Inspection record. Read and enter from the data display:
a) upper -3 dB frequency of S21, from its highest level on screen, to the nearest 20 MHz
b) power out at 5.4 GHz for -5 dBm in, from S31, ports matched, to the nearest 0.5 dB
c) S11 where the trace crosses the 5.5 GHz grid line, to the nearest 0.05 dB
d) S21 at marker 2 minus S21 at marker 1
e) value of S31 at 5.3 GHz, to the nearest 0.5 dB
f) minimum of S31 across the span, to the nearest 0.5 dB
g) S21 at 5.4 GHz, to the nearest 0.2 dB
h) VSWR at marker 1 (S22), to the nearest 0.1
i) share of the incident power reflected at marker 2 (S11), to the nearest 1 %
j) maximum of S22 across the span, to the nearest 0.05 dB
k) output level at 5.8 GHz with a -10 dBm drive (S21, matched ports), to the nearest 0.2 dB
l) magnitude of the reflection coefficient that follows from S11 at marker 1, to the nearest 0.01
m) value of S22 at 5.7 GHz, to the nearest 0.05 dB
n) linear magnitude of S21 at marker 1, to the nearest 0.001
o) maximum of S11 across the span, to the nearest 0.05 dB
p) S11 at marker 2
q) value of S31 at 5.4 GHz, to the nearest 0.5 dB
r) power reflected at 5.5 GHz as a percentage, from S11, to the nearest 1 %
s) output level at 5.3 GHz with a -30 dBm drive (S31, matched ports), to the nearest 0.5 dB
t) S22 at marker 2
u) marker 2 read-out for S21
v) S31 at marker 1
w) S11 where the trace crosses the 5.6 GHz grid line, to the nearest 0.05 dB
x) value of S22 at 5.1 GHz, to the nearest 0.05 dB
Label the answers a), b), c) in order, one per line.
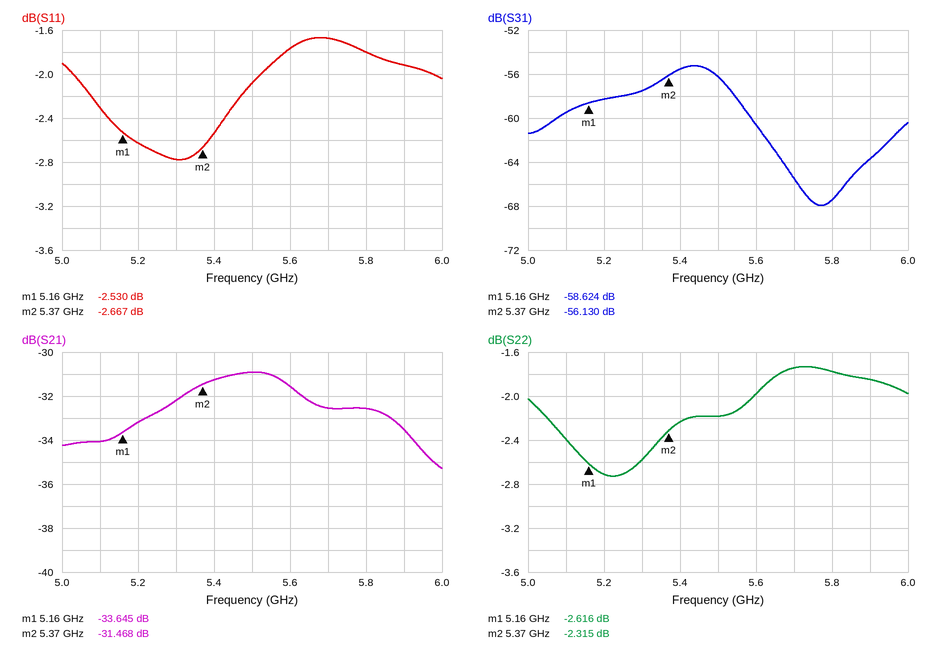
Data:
a) 5.92 GHz
b) -60.5 dBm
c) -2.10 dB
d) 2.177 dB
e) -57.5 dB
f) -68.0 dB
g) -31.2 dB
h) 6.7
i) 54 %
j) -1.75 dB
k) -42.6 dBm
l) 0.75
m) -1.75 dB
n) 0.021
o) -1.65 dB
p) -2.667 dB
q) -55.5 dB
r) 62 %
s) -87.5 dBm
t) -2.315 dB
u) -31.468 dB
v) -58.624 dB
w) -1.75 dB
x) -2.40 dB
